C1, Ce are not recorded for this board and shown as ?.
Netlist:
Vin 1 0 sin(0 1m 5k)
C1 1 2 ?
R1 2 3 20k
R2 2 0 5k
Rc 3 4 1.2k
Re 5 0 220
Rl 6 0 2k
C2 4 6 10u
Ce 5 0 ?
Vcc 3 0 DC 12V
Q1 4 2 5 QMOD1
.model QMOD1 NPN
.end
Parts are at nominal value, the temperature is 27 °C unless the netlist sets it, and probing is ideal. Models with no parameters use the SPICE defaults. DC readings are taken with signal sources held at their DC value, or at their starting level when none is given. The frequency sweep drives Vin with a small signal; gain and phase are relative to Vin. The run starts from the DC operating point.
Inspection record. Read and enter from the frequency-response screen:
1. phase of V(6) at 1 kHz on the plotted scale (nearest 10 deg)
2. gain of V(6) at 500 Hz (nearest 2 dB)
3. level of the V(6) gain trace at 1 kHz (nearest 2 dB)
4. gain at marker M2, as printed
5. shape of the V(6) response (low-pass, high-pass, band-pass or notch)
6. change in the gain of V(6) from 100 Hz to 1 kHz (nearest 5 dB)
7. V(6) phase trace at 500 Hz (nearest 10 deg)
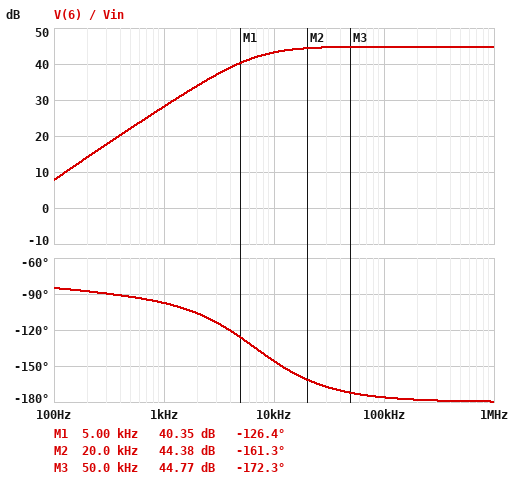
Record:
-100 deg
22 dB
28 dB
44.38 dB
high-pass
20 dB
-90 deg
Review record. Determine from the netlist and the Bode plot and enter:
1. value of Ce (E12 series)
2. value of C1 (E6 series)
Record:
6.8 µF
330 nF
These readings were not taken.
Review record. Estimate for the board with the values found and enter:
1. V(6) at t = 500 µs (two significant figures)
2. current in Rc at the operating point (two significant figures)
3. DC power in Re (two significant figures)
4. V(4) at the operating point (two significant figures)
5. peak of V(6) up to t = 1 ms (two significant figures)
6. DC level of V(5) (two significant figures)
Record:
83 mV
6.0 mA
8.1 mW
4.8 V
100 mV
1.3 V
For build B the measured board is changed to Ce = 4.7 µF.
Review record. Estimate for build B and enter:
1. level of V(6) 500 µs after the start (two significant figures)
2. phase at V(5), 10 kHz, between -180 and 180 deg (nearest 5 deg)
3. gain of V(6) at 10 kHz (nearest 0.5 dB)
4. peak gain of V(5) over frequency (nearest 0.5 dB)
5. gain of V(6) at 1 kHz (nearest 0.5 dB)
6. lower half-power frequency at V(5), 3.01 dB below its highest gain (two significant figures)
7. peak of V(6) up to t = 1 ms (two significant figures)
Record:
73 mV
-45 deg
42.0 dB
-1.5 dB
25.5 dB
120 Hz
83 mV
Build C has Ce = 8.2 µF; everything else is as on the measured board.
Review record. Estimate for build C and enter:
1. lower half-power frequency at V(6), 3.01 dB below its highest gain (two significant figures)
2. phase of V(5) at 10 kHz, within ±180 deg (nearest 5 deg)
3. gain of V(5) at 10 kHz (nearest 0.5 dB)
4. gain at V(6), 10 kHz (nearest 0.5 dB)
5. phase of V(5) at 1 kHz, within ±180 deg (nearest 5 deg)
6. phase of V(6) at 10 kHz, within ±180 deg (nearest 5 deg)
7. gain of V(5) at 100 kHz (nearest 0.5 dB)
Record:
5.8 kHz
-60 deg
-8.0 dB
43.5 dB
-5 deg
-150 deg
-27.0 dB
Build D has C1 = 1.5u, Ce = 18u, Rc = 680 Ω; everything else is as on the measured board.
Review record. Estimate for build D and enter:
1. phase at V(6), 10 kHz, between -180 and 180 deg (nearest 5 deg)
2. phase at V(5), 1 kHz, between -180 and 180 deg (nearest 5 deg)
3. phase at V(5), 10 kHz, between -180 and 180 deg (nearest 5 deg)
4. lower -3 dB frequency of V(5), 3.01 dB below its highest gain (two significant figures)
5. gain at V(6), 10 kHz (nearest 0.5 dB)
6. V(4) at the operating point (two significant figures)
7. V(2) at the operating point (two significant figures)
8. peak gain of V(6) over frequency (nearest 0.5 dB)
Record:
-165 deg
-20 deg
-75 deg
27 Hz
41.0 dB
7.9 V
2.2 V
41.5 dB
